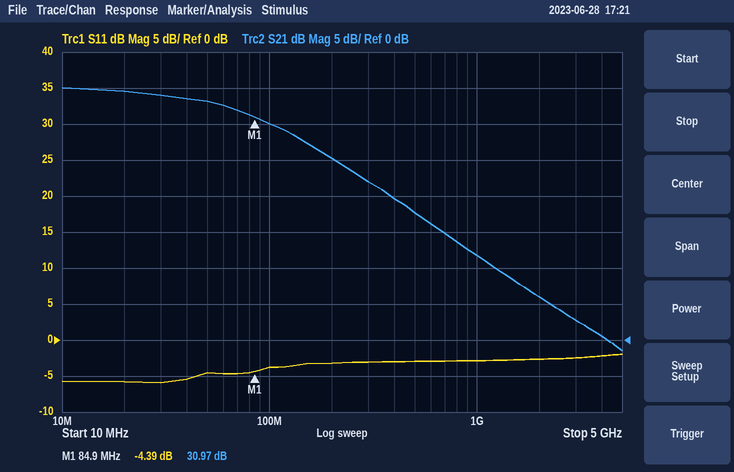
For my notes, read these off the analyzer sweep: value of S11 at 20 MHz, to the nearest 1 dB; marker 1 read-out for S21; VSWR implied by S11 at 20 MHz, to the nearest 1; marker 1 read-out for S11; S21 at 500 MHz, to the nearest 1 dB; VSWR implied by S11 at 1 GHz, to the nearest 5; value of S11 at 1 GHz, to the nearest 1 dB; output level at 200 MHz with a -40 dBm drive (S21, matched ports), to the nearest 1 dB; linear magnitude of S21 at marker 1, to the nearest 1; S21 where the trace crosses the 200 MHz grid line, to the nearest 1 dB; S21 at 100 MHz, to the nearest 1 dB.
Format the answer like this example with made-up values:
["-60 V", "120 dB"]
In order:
["-6 dB", "30.97 dB", "3", "-4.39 dB", "18 dB", "5", "-3 dB", "-15 dBm", "35", "25 dB", "30 dB"]
